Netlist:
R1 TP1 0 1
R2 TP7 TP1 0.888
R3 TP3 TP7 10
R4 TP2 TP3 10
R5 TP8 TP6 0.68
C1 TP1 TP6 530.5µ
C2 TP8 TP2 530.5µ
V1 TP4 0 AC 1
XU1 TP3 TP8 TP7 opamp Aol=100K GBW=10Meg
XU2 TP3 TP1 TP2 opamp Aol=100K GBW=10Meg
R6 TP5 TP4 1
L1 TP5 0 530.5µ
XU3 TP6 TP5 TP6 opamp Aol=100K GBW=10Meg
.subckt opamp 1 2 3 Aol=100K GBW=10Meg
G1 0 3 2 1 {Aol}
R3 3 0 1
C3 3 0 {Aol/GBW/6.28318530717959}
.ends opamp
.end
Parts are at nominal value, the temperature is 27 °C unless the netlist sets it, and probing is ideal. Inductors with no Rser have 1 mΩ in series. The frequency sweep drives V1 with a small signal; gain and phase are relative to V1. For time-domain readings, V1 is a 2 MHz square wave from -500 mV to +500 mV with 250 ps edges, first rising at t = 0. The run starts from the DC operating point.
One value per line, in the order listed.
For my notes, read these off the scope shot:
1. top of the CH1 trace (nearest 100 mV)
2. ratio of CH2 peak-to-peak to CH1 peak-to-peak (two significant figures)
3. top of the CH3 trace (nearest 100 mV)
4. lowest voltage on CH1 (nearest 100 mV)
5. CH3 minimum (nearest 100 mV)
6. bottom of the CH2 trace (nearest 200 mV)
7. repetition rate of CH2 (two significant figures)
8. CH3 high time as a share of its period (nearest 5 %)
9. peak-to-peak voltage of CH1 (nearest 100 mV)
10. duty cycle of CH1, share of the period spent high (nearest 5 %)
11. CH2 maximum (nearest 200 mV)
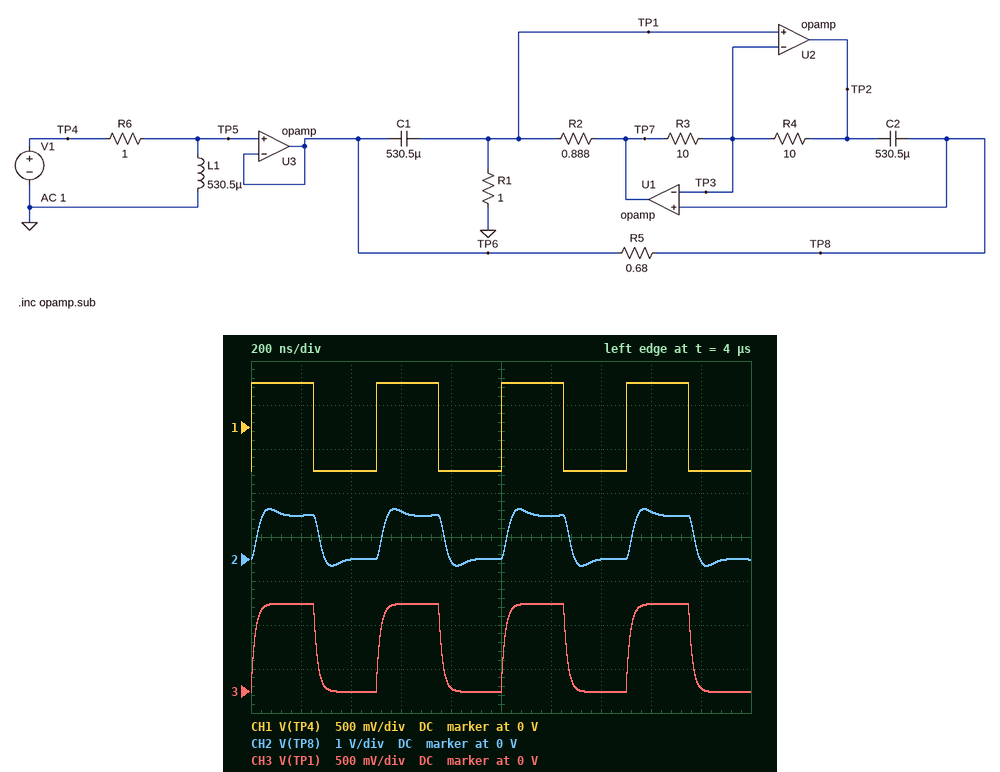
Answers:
500 mV
1.3
1.0 V
-500 mV
0 V
-200 mV
2.0 MHz
50 %
1.0 V
50 %
1.2 V
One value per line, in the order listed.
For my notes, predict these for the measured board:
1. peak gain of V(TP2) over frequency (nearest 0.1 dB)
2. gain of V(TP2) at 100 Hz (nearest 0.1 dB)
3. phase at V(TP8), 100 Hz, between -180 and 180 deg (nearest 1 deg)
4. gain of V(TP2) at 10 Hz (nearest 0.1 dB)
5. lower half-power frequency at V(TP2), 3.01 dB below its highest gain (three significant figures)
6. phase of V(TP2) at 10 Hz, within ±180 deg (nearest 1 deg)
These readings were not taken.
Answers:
0.9 dB
-36.6 dB
59 deg
-48.6 dB
359 Hz
85 deg
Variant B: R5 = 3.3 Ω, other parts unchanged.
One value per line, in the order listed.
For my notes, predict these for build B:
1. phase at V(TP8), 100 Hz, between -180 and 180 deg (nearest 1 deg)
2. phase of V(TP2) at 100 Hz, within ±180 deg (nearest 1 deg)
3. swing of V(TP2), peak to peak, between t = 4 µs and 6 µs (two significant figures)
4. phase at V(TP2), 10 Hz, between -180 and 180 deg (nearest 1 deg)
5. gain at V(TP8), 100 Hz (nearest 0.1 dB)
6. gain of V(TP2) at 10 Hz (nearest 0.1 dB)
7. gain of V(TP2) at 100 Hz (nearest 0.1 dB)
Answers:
16 deg
-164 deg
1.3 V
81 deg
-14.9 dB
-48.8 dB
-24.9 dB
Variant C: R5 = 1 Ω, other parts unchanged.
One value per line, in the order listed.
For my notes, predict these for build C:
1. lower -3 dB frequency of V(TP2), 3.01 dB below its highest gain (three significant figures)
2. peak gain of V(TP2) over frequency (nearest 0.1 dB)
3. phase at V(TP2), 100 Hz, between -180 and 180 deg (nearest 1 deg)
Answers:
324 Hz
0 dB
53 deg
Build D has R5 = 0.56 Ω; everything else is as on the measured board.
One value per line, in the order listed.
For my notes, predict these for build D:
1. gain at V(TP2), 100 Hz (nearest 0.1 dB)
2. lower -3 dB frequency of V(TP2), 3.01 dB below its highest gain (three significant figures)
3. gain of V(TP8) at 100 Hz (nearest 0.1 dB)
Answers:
-34.6 dB
388 Hz
-10.1 dB
